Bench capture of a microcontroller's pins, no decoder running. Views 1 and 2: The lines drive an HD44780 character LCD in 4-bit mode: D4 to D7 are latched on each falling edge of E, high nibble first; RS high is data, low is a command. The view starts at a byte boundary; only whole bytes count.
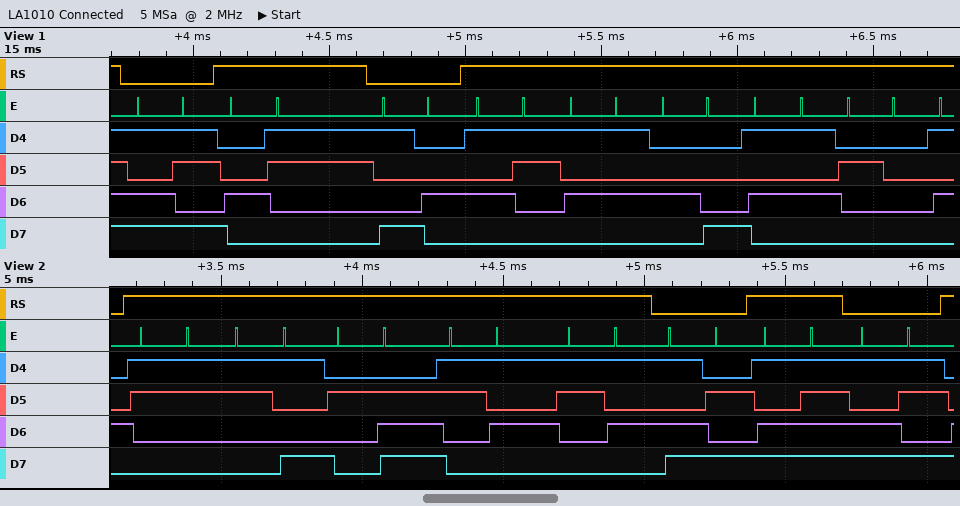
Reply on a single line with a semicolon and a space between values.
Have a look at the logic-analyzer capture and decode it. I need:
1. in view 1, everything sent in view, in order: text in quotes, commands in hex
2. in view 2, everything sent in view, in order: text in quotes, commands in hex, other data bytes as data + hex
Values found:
0xDB "C" 0x94 "SUHU "; "39.55" 0xDA data DF 0xDB
